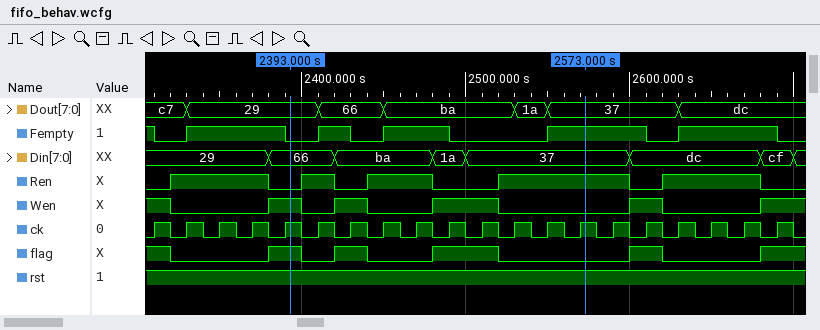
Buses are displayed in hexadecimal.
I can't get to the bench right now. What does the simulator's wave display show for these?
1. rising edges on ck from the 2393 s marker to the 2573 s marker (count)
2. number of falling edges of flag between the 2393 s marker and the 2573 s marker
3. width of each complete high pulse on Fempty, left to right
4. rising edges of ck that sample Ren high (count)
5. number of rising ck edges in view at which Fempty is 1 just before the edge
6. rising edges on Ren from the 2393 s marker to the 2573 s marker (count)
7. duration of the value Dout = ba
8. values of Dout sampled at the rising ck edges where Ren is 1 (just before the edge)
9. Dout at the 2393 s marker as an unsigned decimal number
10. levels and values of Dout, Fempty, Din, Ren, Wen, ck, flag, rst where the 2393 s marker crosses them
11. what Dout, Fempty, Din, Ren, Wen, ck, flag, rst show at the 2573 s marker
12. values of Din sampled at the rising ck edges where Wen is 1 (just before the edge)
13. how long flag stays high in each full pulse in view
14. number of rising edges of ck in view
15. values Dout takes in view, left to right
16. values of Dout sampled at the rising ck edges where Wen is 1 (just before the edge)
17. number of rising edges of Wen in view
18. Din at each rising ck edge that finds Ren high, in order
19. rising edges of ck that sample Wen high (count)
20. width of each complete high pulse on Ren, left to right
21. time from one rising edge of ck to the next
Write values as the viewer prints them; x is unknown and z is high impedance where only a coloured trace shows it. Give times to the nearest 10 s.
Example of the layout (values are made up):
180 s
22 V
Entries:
9
3
60 s, 20 s, 40 s, 60 s, 60 s
13
13
3
80 s
c7, 29, 29, 29, 66, ba, ba, 1a, 37, 37, 37, dc, dc
41
Dout=29, Fempty=0, Din=66, Ren=0, Wen=1, ck=1, flag=1, rst=1
Dout=37, Fempty=1, Din=37, Ren=1, Wen=0, ck=1, flag=0, rst=1
29, 66, ba, 1a, 37, dc, cf
20 s, 20 s, 40 s, 20 s
20
c7, 29, 66, ba, 1a, 37, dc
c7, 29, 66, ba, ba, 37, dc
5
29, 29, 29, 66, ba, ba, 37, 37, 37, 37, dc, dc, dc
7
60 s, 20 s, 40 s, 80 s, 60 s
20 s
